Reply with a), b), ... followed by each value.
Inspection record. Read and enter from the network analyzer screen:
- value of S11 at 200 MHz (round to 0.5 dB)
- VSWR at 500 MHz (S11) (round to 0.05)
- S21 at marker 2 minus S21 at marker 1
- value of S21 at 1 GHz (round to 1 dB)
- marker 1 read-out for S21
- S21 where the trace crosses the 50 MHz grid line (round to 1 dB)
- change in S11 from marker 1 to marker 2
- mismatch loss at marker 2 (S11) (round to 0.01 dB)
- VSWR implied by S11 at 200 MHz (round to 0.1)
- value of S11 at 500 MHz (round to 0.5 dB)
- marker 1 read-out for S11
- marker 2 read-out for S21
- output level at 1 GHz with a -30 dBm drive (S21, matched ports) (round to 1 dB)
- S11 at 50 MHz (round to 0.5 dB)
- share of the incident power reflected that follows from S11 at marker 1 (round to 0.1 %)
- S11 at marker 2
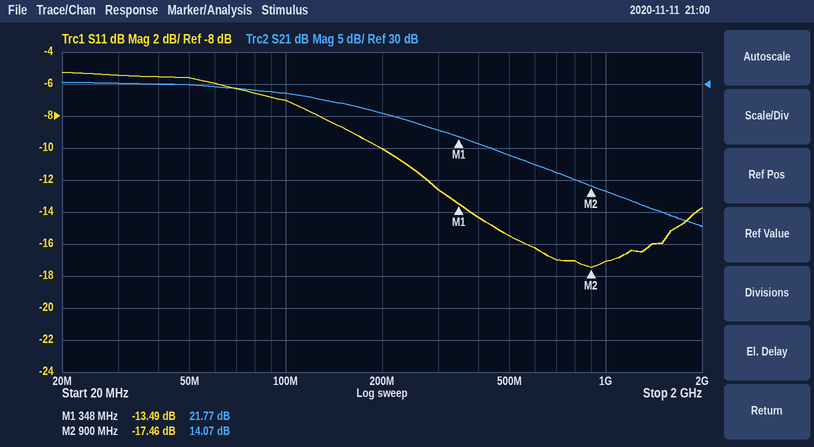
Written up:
a) -10.0 dB
b) 1.40
c) -7.70 dB
d) 13 dB
e) 21.77 dB
f) 30 dB
g) -3.97 dB
h) 0.08 dB
i) 1.9
j) -15.5 dB
k) -13.49 dB
l) 14.07 dB
m) -17 dBm
n) -5.5 dB
o) 4.5 %
p) -17.46 dB
